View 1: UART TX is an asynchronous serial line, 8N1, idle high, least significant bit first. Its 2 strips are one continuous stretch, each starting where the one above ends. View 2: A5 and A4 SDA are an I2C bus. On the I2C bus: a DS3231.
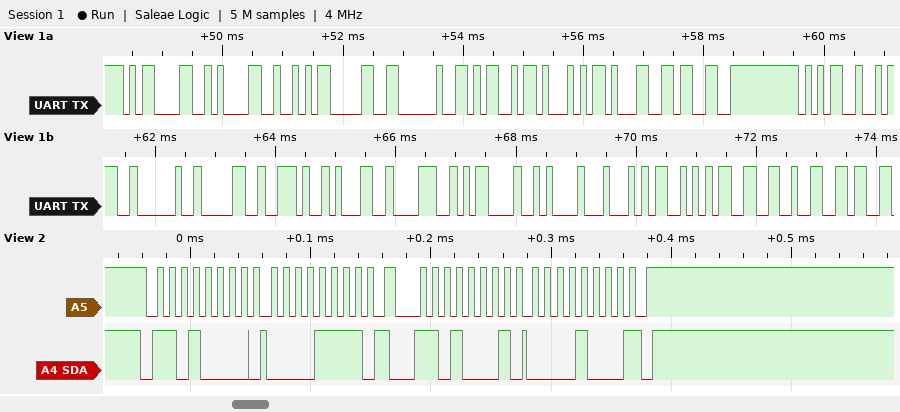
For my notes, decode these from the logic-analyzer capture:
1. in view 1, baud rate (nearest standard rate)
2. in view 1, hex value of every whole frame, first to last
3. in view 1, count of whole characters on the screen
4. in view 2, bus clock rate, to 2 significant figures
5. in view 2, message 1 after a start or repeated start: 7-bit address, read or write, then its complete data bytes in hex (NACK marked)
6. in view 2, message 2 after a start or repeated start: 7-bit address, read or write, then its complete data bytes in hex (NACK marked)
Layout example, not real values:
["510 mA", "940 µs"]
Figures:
["9600 baud", "0x0D 0x0A 0x52 0x30 0x20 0x4D 0x51 0x31 0x33 0x35 0x3A 0x20 0x30 0x2E 0x31 0x38 0x0D 0x0A 0x44 0x53 0x33 0x32", "22", "100 kHz", "0x68 write: 0F", "0x68 read: 08 NACK"]
